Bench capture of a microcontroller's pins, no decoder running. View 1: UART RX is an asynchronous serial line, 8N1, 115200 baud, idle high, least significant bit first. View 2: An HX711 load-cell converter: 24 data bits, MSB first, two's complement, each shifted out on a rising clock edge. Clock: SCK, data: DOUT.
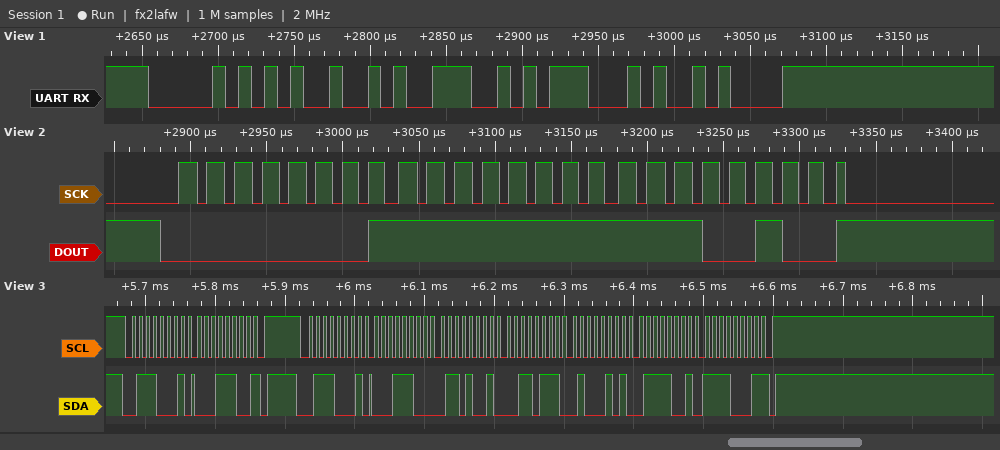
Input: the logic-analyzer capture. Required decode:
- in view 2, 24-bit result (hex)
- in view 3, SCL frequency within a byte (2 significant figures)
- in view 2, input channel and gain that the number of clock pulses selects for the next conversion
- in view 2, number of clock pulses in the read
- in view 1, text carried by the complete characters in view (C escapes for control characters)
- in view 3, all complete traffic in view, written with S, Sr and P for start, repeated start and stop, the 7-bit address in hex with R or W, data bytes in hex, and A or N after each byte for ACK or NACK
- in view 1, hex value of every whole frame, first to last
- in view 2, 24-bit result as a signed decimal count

0x01FFE4
100 kHz
channel A, gain 128
25
"PING\n"
S 38R A 1C N P S 38R A 1C A 69 A 37 A 45 A 79 A F1 N P
0x50 0x49 0x4E 0x47 0x0A
131044
